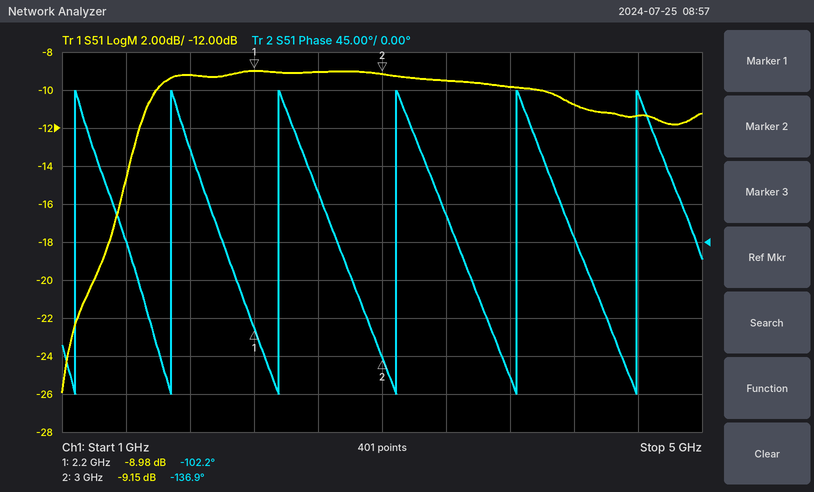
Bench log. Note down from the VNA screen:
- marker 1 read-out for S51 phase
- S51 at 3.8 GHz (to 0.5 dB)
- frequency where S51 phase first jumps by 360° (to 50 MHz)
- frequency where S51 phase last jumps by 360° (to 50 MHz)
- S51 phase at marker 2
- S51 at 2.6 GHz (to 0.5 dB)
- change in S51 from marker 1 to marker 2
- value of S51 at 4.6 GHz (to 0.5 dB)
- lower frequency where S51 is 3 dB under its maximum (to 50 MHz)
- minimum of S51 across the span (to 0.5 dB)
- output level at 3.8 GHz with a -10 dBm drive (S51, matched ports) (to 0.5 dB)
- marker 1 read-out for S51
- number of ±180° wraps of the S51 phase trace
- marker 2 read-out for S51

-102.2°
-10.0 dB
1.10 GHz
4.60 GHz
-136.9°
-9.0 dB
-0.17 dB
-11.5 dB
1.50 GHz
-26.0 dB
-20.0 dBm
-8.98 dB
6
-9.15 dB
